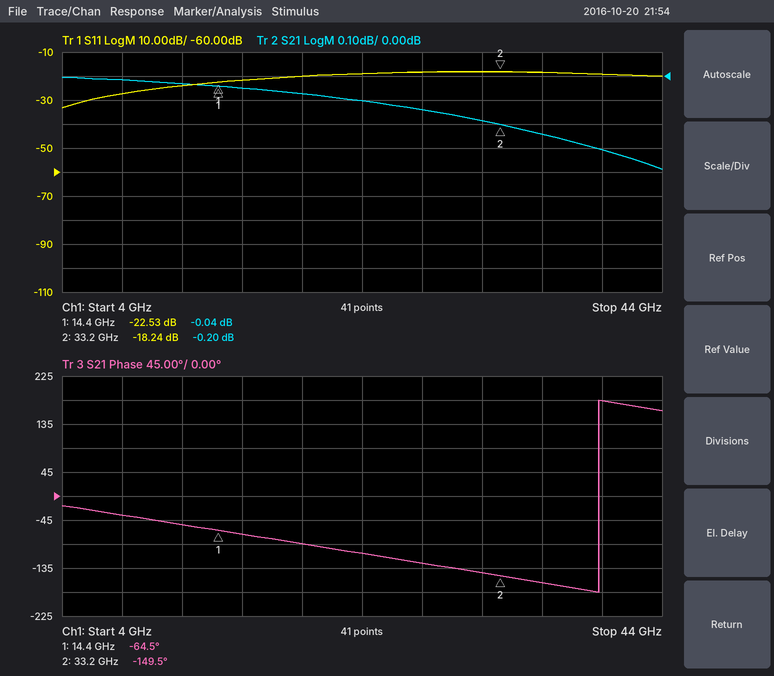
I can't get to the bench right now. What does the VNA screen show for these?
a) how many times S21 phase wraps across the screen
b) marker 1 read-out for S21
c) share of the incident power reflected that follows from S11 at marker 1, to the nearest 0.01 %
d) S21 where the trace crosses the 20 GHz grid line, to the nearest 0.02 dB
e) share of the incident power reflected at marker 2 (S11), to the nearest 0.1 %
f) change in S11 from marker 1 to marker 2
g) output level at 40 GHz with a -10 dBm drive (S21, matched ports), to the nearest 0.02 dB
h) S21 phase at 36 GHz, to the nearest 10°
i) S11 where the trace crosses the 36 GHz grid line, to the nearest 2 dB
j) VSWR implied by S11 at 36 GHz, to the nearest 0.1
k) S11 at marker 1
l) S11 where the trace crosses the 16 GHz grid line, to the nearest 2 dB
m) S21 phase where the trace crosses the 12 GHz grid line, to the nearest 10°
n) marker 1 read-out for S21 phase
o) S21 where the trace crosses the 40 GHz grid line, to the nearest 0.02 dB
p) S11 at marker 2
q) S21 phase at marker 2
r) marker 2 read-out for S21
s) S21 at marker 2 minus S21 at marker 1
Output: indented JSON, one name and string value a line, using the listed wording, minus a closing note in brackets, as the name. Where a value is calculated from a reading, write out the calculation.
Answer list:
{
  "how many times S21 phase wraps across the screen": "1",
  "marker 1 read-out for S21": "-0.04 dB",
  "share of the incident power reflected that follows from S11 at marker 1, to the nearest 0.01 %": "10^(-22.53/10) ≈ 0.56 %",
  "S21 where the trace crosses the 20 GHz grid line, to the nearest 0.02 dB": "-0.08 dB",
  "share of the incident power reflected at marker 2 (S11), to the nearest 0.1 %": "10^(-18.24/10) ≈ 1.5 %",
  "change in S11 from marker 1 to marker 2": "-18.24 − (-22.53) = 4.29 dB",
  "output level at 40 GHz with a -10 dBm drive (S21, matched ports), to the nearest 0.02 dB": "-10 dBm + (-0.30 dB) = -10.30 dBm",
  "S21 phase at 36 GHz, to the nearest 10°": "-160°",
  "S11 where the trace crosses the 36 GHz grid line, to the nearest 2 dB": "-18 dB",
  "VSWR implied by S11 at 36 GHz, to the nearest 0.1": "|Γ| = 10^(-18/20) = 0.1259; VSWR = (1 + 0.1259)/(1 − 0.1259) ≈ 1.3",
  "S11 at marker 1": "-22.53 dB",
  "S11 where the trace crosses the 16 GHz grid line, to the nearest 2 dB": "-22 dB",
  "S21 phase where the trace crosses the 12 GHz grid line, to the nearest 10°": "-50°",
  "marker 1 read-out for S21 phase": "-64.5°",
  "S21 where the trace crosses the 40 GHz grid line, to the nearest 0.02 dB": "-0.30 dB",
  "S11 at marker 2": "-18.24 dB",
  "S21 phase at marker 2": "-149.5°",
  "marker 2 read-out for S21": "-0.20 dB",
  "S21 at marker 2 minus S21 at marker 1": "-0.2 − (-0.04) = -0.16 dB"
}
